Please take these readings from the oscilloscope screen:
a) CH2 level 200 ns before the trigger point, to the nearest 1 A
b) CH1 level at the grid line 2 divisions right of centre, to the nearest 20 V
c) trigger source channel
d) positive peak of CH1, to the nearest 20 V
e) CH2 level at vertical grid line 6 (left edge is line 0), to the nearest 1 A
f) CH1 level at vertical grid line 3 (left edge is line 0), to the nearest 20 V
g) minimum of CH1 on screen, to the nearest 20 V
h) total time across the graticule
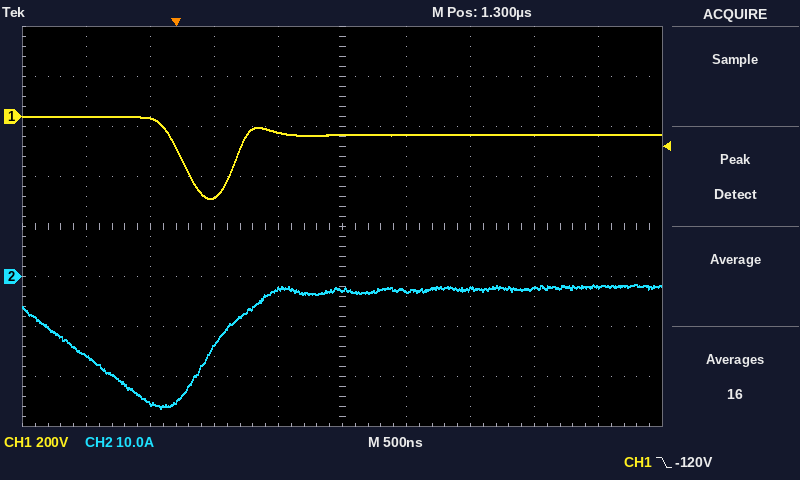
-25 A
-80 V
CH1
0 V
-3 A
-320 V
-320 V
5 µs
